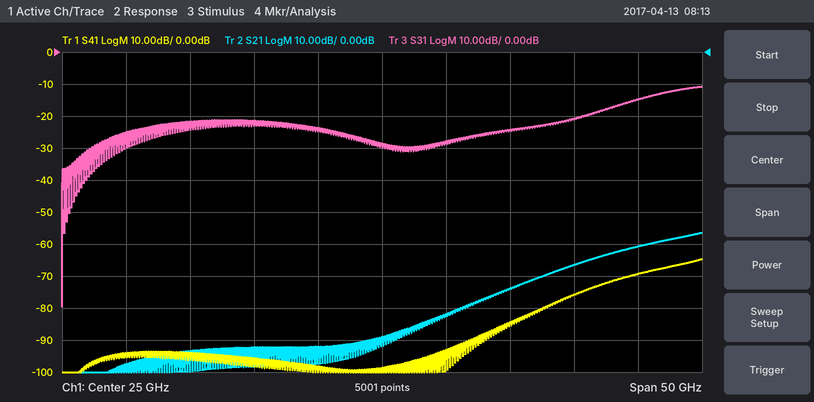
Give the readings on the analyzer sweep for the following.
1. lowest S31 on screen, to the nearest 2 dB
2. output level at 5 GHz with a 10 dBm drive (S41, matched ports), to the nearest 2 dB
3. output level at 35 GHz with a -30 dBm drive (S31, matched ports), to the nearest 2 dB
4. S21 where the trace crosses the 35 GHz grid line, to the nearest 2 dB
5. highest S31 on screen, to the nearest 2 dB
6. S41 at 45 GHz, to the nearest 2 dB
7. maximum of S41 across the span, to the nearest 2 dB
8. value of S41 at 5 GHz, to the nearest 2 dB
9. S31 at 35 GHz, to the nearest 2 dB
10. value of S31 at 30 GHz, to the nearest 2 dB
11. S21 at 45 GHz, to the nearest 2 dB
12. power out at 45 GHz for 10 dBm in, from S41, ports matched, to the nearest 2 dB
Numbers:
-80 dB
-84 dBm
-54 dBm
-74 dB
-10 dB
-70 dB
-64 dB
-94 dB
-24 dB
-28 dB
-60 dB
-60 dBm
